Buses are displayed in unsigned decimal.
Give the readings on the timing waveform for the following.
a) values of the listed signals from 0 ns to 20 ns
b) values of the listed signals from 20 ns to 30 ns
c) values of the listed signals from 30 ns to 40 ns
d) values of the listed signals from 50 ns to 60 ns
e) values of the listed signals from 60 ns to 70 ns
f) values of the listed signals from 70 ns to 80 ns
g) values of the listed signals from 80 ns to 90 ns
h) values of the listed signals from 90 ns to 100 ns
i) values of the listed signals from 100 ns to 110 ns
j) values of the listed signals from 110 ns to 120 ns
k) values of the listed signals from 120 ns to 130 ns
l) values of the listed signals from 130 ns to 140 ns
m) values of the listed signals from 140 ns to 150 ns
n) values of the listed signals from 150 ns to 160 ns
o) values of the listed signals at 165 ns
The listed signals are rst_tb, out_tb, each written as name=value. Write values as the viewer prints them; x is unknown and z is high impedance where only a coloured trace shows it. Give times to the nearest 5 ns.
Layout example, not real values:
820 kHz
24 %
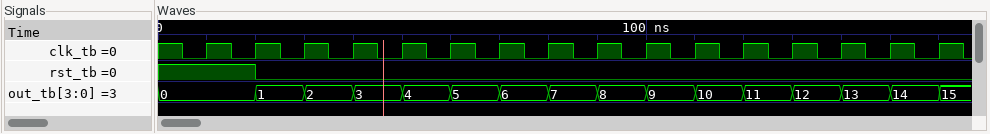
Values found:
rst_tb=1, out_tb=0
rst_tb=0, out_tb=1
rst_tb=0, out_tb=2
rst_tb=0, out_tb=4
rst_tb=0, out_tb=5
rst_tb=0, out_tb=6
rst_tb=0, out_tb=7
rst_tb=0, out_tb=8
rst_tb=0, out_tb=9
rst_tb=0, out_tb=10
rst_tb=0, out_tb=11
rst_tb=0, out_tb=12
rst_tb=0, out_tb=13
rst_tb=0, out_tb=14
rst_tb=0, out_tb=15
